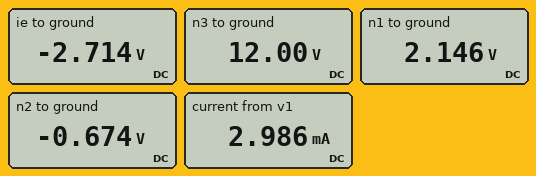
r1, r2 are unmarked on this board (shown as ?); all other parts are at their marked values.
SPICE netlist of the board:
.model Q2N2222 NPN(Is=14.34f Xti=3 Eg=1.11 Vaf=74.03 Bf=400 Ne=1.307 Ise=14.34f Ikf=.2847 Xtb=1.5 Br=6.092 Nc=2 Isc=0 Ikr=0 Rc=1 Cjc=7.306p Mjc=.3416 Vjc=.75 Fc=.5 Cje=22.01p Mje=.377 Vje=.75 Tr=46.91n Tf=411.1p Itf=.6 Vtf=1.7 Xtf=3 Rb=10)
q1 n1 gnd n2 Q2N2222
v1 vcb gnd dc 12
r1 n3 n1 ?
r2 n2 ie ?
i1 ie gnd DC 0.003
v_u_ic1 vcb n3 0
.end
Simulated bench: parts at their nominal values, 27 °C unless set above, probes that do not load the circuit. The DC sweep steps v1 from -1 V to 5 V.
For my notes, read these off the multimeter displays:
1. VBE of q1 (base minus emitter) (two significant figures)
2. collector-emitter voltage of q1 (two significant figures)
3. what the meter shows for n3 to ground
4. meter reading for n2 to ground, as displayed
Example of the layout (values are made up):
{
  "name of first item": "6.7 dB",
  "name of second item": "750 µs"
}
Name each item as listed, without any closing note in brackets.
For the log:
{
  "VBE of q1 (base minus emitter)": "670 mV",
  "collector-emitter voltage of q1": "2.8 V",
  "what the meter shows for n3 to ground": "12.00 V",
  "meter reading for n2 to ground, as displayed": "-0.674 V"
}
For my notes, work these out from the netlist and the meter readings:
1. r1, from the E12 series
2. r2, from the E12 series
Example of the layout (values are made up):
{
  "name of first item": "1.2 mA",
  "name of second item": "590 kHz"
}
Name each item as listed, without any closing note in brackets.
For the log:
{
  "r1, from the E12 series": "3.3 kΩ",
  "r2, from the E12 series": "680 Ω"
}
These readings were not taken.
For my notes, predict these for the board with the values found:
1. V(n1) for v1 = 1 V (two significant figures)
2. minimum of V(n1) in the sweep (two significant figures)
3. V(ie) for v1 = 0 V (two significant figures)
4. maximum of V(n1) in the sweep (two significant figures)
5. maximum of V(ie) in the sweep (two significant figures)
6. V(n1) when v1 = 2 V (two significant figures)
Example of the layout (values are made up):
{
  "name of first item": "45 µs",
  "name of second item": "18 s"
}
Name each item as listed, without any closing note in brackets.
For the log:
{
  "V(n1) for v1 = 1 V": "-740 mV",
  "minimum of V(n1) in the sweep": "-750 mV",
  "V(ie) for v1 = 0 V": "-2.8 V",
  "maximum of V(n1) in the sweep": "-710 mV",
  "maximum of V(ie) in the sweep": "-2.8 V",
  "V(n1) when v1 = 2 V": "-730 mV"
}
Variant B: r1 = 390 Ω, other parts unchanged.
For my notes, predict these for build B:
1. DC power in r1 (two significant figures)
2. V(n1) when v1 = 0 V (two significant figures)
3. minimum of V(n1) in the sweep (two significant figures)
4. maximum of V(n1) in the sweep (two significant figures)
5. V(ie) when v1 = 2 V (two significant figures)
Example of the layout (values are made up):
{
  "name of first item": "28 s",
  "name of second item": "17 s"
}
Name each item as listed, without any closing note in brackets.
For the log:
{
  "DC power in r1": "3.5 mW",
  "V(n1) when v1 = 0 V": "-710 mV",
  "minimum of V(n1) in the sweep": "-760 mV",
  "maximum of V(n1) in the sweep": "3.8 V",
  "V(ie) when v1 = 2 V": "-2.7 V"
}
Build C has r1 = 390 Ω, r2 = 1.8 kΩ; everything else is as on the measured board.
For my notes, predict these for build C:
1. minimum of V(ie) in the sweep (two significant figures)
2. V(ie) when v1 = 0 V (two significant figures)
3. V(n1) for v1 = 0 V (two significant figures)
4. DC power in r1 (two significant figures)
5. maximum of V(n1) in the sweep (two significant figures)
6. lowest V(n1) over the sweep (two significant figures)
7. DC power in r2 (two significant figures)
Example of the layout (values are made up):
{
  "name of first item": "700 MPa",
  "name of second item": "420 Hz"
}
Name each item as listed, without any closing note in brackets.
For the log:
{
  "minimum of V(ie) in the sweep": "-6.2 V",
  "V(ie) when v1 = 0 V": "-6.1 V",
  "V(n1) for v1 = 0 V": "-710 mV",
  "DC power in r1": "3.5 mW",
  "maximum of V(n1) in the sweep": "3.8 V",
  "lowest V(n1) over the sweep": "-760 mV",
  "DC power in r2": "16 mW"
}
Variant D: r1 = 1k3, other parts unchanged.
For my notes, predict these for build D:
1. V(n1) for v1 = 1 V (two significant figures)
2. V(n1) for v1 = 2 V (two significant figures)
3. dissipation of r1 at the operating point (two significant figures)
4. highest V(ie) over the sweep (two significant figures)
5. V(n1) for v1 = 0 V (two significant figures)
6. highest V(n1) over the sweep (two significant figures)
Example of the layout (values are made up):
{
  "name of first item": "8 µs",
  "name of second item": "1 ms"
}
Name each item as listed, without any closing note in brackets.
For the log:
{
  "V(n1) for v1 = 1 V": "-720 mV",
  "V(n1) for v1 = 2 V": "-700 mV",
  "dissipation of r1 at the operating point": "12 mW",
  "highest V(ie) over the sweep": "-2.7 V",
  "V(n1) for v1 = 0 V": "-740 mV",
  "highest V(n1) over the sweep": "1.1 V"
}
